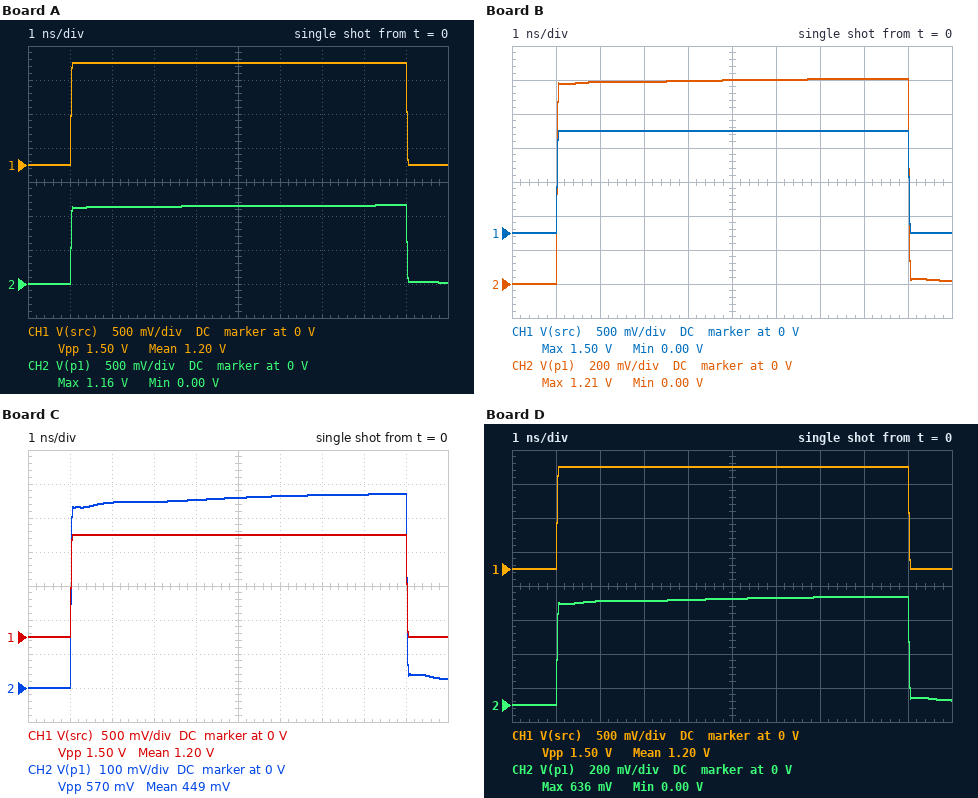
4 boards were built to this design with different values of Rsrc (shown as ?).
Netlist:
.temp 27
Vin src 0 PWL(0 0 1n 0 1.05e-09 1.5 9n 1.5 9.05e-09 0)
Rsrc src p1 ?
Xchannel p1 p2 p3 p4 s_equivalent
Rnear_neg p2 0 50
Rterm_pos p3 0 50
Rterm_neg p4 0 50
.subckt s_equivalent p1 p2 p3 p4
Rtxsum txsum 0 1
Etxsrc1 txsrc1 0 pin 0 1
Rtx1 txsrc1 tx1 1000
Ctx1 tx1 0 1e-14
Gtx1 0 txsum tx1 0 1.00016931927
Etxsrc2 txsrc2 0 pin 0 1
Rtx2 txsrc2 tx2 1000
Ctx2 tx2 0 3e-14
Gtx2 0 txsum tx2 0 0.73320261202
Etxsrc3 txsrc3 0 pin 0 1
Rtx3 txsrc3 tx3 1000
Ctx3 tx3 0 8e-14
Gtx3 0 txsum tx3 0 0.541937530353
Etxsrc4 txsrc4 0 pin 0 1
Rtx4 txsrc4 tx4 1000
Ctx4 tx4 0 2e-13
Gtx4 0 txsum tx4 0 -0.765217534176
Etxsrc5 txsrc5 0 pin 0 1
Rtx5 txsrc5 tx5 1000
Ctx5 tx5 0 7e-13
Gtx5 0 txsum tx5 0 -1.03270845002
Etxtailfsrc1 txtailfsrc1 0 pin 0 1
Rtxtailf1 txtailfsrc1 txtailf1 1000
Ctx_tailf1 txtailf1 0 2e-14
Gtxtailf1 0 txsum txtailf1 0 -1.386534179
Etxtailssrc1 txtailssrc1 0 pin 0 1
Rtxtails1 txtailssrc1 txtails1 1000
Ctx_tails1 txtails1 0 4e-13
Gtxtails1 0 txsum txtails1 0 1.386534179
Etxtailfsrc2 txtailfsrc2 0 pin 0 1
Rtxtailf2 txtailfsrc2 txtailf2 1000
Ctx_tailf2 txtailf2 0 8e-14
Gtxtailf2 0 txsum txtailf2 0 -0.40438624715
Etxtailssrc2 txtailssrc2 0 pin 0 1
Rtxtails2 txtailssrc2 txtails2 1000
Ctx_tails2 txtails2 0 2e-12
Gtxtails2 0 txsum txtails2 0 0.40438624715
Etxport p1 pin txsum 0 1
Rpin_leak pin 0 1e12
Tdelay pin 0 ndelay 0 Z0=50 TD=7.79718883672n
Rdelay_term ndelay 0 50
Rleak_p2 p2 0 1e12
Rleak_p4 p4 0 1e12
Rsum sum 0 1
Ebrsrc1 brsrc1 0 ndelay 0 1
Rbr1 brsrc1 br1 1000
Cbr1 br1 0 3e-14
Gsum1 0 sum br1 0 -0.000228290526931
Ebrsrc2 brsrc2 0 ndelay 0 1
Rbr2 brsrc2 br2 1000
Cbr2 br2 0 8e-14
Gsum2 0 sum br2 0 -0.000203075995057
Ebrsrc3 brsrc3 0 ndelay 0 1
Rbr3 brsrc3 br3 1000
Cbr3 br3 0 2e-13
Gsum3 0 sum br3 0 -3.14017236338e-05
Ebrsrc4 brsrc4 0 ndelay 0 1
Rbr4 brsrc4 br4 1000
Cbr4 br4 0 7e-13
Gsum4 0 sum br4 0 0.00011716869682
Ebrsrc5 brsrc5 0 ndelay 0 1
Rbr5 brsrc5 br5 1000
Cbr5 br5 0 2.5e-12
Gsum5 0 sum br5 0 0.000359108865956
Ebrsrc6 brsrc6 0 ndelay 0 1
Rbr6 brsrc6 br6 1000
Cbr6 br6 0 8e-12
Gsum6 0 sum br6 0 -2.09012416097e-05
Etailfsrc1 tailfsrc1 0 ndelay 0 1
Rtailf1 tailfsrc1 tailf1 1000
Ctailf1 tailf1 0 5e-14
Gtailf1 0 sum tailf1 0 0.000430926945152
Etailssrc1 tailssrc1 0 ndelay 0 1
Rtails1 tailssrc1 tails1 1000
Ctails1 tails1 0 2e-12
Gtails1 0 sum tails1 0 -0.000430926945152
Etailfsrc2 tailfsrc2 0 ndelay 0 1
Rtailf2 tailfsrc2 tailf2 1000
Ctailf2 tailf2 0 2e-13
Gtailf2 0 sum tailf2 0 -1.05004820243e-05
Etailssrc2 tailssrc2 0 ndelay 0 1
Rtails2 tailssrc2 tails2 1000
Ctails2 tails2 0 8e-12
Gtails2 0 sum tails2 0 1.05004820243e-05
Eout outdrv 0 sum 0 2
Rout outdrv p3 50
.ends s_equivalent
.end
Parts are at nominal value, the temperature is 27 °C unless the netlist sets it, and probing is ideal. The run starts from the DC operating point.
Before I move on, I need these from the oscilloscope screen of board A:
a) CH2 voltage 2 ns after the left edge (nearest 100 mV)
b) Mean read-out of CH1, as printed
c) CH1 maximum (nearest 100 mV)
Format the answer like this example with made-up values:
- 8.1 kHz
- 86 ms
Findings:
- 1.1 V
- 1.20 V
- 1.5 V
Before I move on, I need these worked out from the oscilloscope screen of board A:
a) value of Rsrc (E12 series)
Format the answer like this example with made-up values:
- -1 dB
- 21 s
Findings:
- 22 Ω
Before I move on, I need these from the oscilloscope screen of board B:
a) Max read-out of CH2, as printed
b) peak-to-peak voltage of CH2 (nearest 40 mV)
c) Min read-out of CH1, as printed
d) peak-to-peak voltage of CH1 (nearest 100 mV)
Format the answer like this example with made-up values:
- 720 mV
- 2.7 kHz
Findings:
- 1.21 V
- 1.20 V
- 0.00 V
- 1.5 V
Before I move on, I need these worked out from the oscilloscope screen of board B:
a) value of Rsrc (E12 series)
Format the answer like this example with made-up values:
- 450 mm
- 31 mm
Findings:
- 18 Ω
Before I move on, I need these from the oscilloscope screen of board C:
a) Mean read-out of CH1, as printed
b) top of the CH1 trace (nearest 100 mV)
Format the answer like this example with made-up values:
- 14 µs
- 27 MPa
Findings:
- 1.20 V
- 1.5 V
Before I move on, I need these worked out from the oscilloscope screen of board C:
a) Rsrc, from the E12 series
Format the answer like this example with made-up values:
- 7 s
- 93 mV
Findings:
- 120 Ω
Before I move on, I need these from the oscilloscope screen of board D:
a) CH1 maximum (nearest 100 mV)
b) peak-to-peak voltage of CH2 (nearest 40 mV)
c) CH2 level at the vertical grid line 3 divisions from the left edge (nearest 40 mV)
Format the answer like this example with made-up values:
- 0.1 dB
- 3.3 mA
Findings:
- 1.5 V
- 640 mV
- 600 mV
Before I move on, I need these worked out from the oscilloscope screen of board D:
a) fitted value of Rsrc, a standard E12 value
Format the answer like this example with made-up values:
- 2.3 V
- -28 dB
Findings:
- 100 Ω
